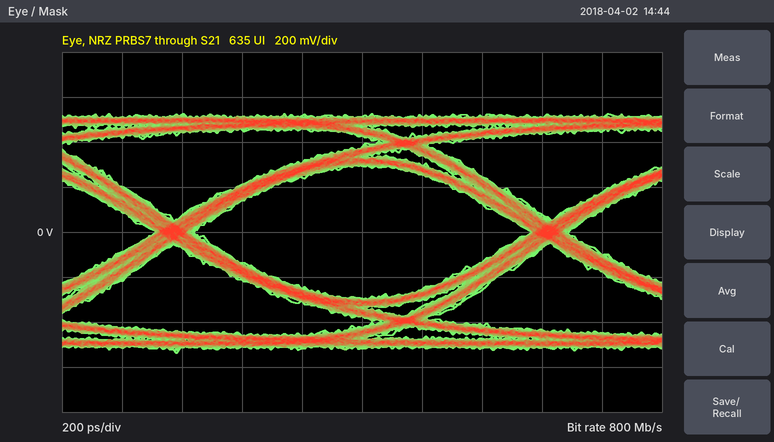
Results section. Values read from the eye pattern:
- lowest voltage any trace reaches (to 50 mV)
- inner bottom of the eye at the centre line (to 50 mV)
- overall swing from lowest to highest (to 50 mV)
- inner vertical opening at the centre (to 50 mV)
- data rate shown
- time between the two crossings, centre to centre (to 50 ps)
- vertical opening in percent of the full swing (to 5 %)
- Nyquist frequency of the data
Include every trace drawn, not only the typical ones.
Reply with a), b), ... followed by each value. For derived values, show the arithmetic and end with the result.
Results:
a) -550 mV
b) -300 mV
c) 1.05 V
d) 600 mV
e) 800 Mb/s
f) 1.25 ns
g) 600 mV / 1.05 V ≈ 57.1 %, so 55 % to the nearest 5 %
h) 400 MHz
